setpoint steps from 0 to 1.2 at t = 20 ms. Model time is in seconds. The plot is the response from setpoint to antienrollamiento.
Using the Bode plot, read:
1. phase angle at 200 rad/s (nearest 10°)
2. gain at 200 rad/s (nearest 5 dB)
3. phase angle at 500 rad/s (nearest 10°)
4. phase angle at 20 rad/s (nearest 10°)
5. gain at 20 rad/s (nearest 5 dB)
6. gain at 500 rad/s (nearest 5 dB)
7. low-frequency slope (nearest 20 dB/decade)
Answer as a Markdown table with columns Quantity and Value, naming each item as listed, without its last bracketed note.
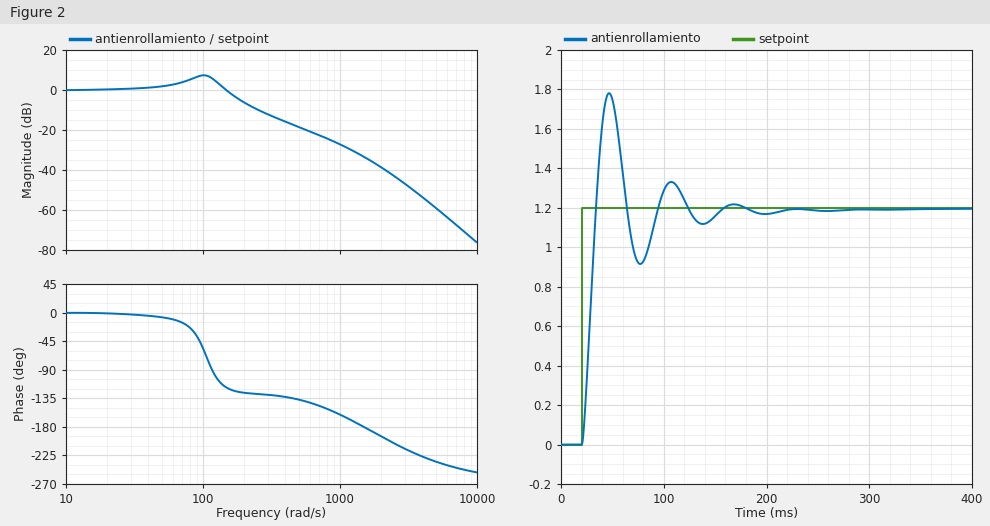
| Quantity | Value |
|---|---|
| phase angle at 200 rad/s | -130° |
| gain at 200 rad/s | -5 dB |
| phase angle at 500 rad/s | -140° |
| phase angle at 20 rad/s | 0° |
| gain at 20 rad/s | 0 dB |
| gain at 500 rad/s | -20 dB |
| low-frequency slope | 0 dB/decade |
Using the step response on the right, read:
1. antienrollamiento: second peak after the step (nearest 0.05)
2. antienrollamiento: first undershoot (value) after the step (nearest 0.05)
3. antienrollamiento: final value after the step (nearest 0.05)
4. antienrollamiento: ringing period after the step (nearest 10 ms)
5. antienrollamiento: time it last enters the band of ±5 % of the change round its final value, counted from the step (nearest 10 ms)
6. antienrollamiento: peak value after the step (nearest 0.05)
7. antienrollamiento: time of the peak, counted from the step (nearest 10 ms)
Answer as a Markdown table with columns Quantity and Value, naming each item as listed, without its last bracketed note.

| Quantity | Value |
|---|---|
| antienrollamiento: second peak after the step | 1.35 |
| antienrollamiento: first undershoot (value) after the step | 0.90 |
| antienrollamiento: final value after the step | 1.20 |
| antienrollamiento: ringing period after the step | 60 ms |
| antienrollamiento: time it last enters the band of ±5 % of the change round its final value, counted from the step | 130 ms |
| antienrollamiento: peak value after the step | 1.80 |
| antienrollamiento: time of the peak, counted from the step | 30 ms |
